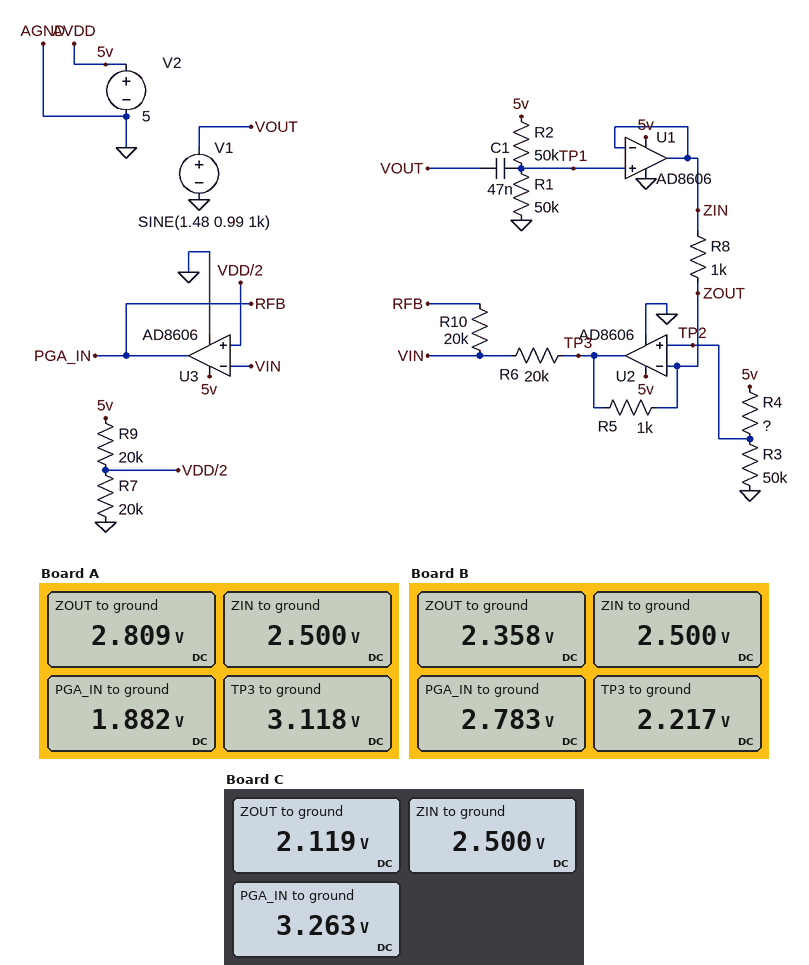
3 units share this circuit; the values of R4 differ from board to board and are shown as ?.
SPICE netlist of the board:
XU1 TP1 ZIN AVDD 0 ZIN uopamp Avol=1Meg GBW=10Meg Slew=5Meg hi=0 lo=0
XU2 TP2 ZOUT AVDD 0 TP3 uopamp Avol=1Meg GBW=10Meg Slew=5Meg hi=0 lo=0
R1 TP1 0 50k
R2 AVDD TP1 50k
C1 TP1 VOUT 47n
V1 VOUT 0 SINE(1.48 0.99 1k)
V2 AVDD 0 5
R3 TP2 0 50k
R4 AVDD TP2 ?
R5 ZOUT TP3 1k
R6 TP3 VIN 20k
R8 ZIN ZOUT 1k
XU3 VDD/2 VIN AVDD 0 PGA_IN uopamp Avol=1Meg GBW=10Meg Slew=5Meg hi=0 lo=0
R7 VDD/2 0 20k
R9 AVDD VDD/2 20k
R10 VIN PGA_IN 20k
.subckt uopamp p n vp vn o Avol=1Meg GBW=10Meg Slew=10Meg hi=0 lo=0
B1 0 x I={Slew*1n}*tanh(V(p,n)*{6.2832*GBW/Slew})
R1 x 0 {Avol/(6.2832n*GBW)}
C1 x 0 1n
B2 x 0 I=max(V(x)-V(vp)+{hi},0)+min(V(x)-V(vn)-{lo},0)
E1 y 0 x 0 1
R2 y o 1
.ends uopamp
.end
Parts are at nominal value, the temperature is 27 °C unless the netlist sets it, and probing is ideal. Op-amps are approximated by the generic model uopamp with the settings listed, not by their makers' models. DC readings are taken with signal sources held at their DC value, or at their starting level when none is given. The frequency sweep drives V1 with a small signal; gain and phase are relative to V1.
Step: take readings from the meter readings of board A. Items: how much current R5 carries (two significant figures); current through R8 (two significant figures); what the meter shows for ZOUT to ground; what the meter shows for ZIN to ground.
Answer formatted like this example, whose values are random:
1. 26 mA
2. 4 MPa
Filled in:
1. 310 µA
2. 310 µA
3. 2.809 V
4. 2.500 V
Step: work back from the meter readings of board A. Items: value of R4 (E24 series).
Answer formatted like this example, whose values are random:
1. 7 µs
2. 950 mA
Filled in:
1. 39 kΩ
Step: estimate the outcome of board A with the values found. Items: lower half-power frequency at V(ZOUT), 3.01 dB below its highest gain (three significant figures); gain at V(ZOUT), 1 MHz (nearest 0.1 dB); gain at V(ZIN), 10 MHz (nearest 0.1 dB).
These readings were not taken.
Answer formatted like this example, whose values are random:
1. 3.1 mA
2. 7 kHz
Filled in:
1. 2.81 MHz
2. -20.2 dB
3. -3.0 dB
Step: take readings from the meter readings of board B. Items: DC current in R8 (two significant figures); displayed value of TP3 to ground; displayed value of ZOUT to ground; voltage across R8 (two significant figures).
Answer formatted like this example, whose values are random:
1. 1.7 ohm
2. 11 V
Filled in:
1. 140 µA
2. 2.217 V
3. 2.358 V
4. 140 mV
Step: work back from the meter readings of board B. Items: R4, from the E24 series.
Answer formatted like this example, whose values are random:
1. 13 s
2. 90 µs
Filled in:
1. 56 kΩ
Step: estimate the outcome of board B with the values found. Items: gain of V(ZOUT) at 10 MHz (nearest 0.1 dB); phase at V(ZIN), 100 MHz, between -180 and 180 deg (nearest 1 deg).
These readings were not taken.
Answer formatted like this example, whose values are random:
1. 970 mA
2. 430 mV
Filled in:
1. -10.0 dB
2. -84 deg
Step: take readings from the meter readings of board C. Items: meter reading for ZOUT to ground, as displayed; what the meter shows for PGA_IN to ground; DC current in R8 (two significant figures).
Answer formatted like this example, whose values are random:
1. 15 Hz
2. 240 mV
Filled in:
1. 2.119 V
2. 3.263 V
3. 380 µA
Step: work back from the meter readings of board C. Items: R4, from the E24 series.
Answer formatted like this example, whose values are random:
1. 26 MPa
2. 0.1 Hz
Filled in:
1. 68 kΩ
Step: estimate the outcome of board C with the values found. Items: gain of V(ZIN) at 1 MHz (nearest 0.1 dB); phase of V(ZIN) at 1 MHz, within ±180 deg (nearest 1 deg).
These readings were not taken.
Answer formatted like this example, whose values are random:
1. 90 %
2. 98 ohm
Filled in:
1. 0 dB
2. -6 deg
